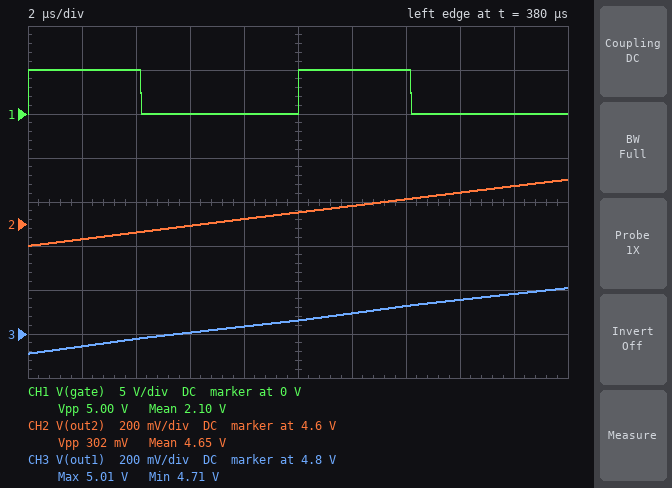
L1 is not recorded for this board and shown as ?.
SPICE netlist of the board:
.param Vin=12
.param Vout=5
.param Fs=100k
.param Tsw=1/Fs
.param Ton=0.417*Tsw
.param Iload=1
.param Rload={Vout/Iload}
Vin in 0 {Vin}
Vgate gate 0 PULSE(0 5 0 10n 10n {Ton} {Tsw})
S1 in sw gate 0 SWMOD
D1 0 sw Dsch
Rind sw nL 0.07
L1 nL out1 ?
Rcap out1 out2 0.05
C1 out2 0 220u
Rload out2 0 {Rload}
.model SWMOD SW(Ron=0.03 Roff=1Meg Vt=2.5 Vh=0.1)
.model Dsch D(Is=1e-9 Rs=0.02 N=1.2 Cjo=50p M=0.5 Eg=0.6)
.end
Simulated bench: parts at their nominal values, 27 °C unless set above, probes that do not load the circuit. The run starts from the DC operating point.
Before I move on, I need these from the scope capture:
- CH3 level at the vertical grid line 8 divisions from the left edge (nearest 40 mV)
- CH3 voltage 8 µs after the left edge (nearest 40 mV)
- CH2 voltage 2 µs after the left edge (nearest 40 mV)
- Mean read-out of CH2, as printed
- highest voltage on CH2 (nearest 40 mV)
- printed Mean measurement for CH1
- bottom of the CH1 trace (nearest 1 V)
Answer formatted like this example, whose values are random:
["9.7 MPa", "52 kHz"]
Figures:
["4.96 V", "4.84 V", "4.52 V", "4.65 V", "4.80 V", "2.10 V", "0 V"]
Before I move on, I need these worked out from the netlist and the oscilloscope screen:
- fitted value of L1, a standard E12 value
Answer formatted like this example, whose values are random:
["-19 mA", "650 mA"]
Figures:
["220 µH"]
